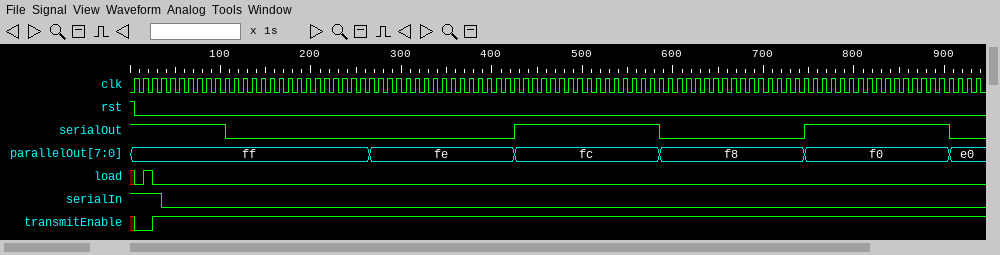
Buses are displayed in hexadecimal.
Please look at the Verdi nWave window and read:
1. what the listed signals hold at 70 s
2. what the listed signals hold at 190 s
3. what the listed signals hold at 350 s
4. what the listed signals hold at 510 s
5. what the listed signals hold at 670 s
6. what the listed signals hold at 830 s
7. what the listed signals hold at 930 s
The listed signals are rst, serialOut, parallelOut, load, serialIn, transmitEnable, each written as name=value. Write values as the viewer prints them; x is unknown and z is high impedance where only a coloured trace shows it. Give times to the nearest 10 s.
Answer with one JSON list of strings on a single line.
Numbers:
["rst=0, serialOut=1, parallelOut=ff, load=0, serialIn=0, transmitEnable=1", "rst=0, serialOut=0, parallelOut=ff, load=0, serialIn=0, transmitEnable=1", "rst=0, serialOut=0, parallelOut=fe, load=0, serialIn=0, transmitEnable=1", "rst=0, serialOut=1, parallelOut=fc, load=0, serialIn=0, transmitEnable=1", "rst=0, serialOut=0, parallelOut=f8, load=0, serialIn=0, transmitEnable=1", "rst=0, serialOut=1, parallelOut=f0, load=0, serialIn=0, transmitEnable=1", "rst=0, serialOut=0, parallelOut=e0, load=0, serialIn=0, transmitEnable=1"]
